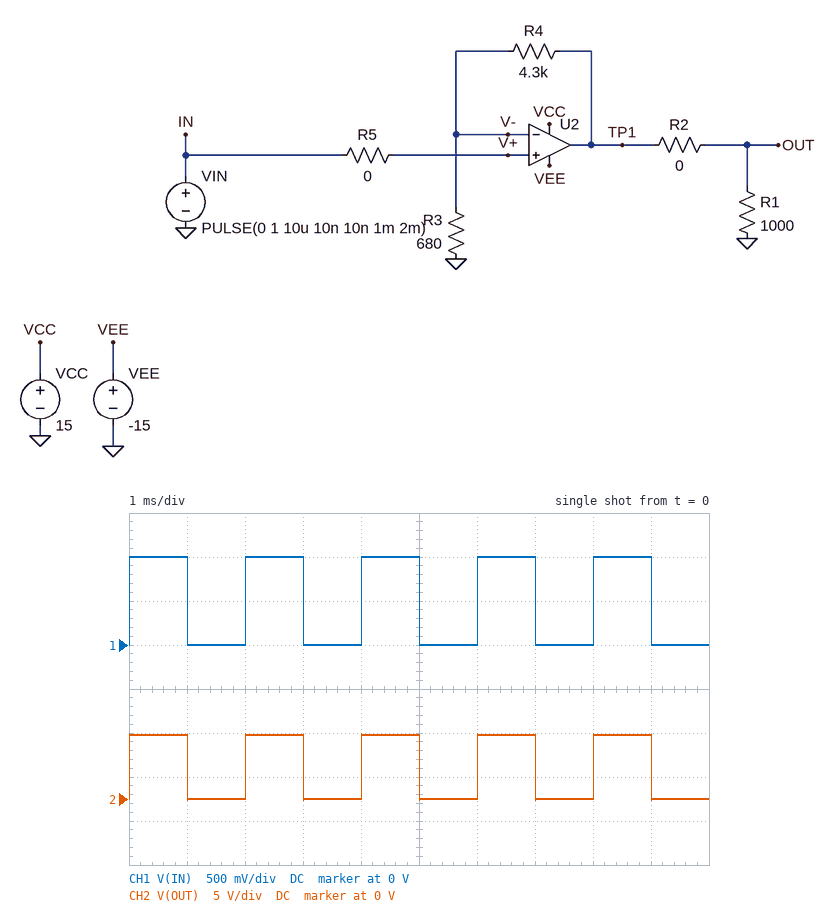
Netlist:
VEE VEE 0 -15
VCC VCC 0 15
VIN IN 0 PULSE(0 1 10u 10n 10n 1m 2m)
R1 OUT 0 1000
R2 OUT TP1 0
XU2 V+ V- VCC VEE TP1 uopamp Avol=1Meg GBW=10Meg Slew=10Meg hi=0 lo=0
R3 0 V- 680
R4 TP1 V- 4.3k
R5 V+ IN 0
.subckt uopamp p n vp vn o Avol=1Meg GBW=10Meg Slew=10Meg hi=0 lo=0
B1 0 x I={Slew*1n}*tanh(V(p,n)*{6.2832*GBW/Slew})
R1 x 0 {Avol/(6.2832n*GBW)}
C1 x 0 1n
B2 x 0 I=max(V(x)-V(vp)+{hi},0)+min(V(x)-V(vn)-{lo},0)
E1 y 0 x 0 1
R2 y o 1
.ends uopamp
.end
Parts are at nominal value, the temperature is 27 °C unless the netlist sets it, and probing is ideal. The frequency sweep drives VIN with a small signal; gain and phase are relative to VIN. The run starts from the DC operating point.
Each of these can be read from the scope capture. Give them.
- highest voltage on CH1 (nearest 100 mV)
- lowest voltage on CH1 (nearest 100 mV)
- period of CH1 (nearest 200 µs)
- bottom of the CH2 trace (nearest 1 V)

1.0 V
0 V
2.0 ms
0 V
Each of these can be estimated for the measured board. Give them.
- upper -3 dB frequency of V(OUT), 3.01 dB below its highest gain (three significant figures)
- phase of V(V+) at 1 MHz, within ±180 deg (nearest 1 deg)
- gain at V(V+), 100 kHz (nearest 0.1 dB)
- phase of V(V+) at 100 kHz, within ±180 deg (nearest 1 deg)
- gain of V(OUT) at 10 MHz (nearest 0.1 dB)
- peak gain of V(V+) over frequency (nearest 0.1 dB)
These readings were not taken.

1.36 MHz
0 deg
0 dB
0 deg
-0.1 dB
0 dB
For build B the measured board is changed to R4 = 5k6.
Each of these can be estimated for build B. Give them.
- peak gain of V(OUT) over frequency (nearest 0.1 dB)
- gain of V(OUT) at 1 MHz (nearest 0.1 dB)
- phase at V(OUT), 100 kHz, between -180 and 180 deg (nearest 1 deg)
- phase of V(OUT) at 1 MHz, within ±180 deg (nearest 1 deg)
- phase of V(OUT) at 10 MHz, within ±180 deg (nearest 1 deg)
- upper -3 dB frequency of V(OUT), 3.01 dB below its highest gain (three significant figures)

19.3 dB
16.6 dB
-5 deg
-43 deg
-84 deg
1.08 MHz
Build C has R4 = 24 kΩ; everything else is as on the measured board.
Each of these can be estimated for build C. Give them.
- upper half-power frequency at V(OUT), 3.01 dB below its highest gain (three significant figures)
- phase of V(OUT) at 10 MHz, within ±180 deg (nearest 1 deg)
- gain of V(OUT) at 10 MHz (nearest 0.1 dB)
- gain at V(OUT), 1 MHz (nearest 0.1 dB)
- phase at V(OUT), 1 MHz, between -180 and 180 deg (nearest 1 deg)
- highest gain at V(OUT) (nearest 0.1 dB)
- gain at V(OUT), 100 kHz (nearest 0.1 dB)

275 kHz
-88 deg
0 dB
19.7 dB
-75 deg
31.2 dB
30.7 dB
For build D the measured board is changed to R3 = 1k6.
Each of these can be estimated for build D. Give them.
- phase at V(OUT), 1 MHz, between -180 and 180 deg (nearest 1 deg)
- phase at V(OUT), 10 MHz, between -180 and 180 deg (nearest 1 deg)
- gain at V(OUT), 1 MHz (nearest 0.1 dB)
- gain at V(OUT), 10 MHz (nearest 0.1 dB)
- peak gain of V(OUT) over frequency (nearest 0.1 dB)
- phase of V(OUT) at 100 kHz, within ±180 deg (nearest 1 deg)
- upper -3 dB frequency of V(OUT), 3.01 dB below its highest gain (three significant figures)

-20 deg
-75 deg
10.8 dB
-0.3 dB
11.3 dB
-2 deg
2.71 MHz
